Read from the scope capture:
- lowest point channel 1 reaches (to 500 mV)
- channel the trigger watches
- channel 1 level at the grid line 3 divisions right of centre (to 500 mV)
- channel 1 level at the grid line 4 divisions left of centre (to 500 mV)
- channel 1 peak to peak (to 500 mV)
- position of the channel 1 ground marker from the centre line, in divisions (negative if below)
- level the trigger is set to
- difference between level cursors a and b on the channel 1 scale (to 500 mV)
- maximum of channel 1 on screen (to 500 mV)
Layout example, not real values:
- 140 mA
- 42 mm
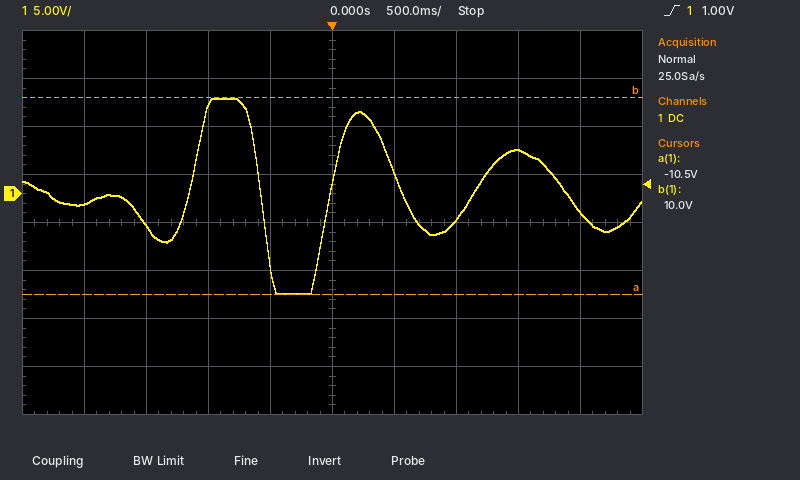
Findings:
- -10.5 V
- channel 1
- 4.5 V
- -1.0 V
- 20.5 V
- +0.6 div
- 1.00 V
- 20.5 V
- 10.0 V
